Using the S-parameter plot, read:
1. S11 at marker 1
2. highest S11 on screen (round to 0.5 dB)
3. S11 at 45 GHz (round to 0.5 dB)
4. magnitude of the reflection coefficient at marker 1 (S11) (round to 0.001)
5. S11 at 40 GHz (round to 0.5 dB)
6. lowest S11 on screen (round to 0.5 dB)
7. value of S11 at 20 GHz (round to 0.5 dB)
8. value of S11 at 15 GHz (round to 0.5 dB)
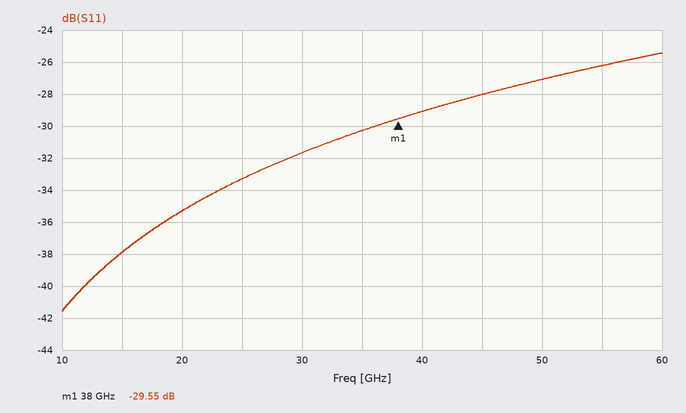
-29.55 dB
-25.5 dB
-28.0 dB
0.033
-29.0 dB
-41.5 dB
-35.5 dB
-38.0 dB
